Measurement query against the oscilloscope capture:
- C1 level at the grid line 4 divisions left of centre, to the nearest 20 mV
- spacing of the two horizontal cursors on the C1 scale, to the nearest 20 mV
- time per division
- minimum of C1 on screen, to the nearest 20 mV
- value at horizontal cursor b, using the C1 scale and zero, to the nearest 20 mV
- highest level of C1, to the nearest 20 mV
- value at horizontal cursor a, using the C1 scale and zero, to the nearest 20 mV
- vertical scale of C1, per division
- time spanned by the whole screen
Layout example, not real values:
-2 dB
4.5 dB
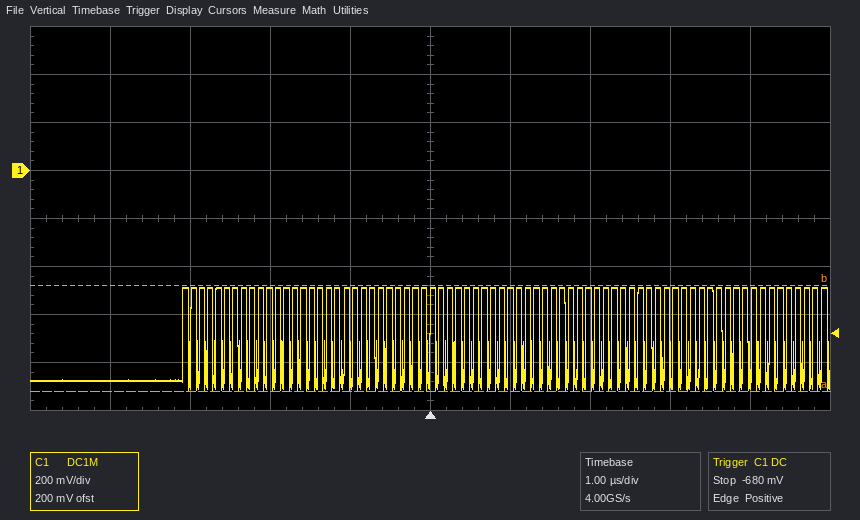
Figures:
-880 mV
440 mV
1 µs
-920 mV
-480 mV
-480 mV
-920 mV
200 mV
10 µs
